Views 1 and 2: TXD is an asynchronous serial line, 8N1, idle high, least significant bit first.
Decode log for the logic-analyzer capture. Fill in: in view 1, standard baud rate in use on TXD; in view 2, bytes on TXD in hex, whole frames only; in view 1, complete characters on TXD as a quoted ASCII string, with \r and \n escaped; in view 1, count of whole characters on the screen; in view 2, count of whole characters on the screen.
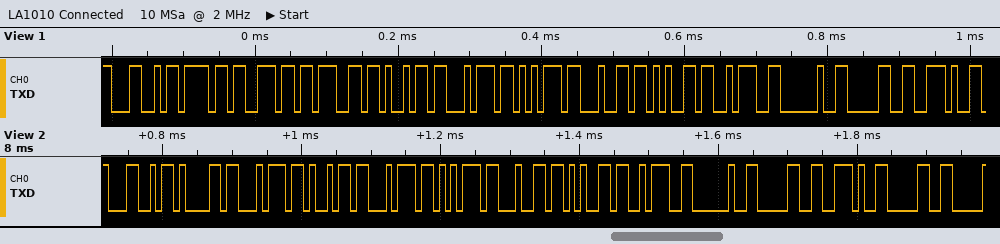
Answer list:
115200 baud
4C 61 74 69 74 75 64 65 3A 20 30 2E 30
"Longitude: 0."
13
13
